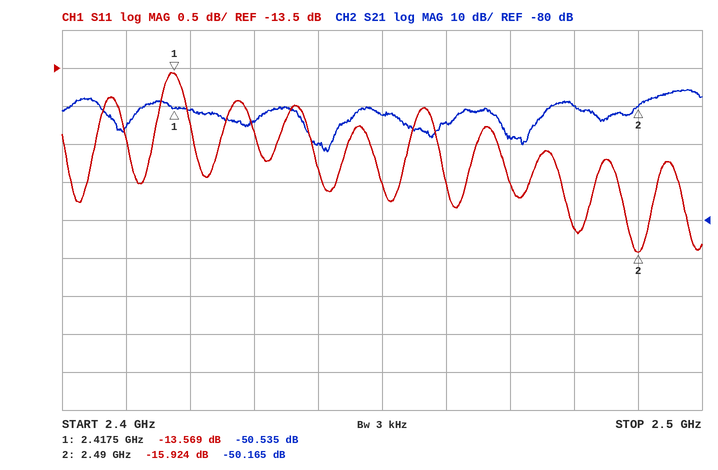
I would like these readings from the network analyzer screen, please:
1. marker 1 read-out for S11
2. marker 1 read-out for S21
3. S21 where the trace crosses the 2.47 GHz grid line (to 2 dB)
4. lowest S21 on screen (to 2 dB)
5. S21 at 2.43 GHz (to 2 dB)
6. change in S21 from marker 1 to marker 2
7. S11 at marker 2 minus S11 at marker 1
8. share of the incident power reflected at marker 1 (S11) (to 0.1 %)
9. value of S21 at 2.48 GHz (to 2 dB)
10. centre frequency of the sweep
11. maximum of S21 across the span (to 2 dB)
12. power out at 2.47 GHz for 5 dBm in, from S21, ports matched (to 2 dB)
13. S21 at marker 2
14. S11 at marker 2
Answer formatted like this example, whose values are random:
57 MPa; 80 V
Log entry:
-13.569 dB; -50.535 dB; -58 dB; -62 dB; -54 dB; 0.370 dB; -2.355 dB; 4.4 %; -50 dB; 2.45 GHz; -46 dB; -54 dBm; -50.165 dB; -15.924 dB
